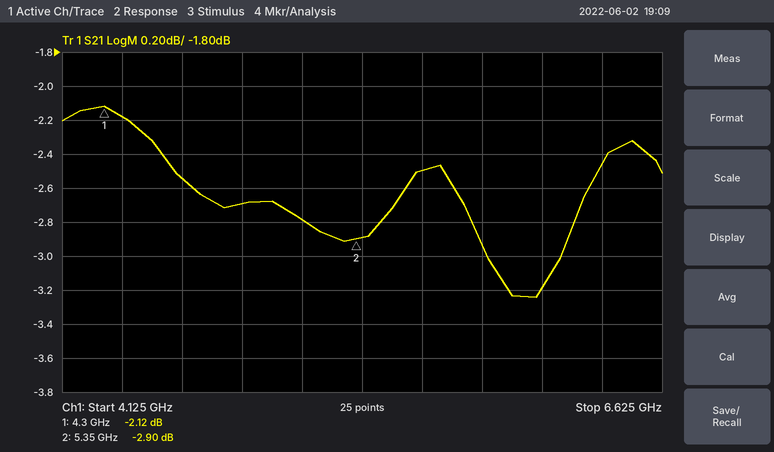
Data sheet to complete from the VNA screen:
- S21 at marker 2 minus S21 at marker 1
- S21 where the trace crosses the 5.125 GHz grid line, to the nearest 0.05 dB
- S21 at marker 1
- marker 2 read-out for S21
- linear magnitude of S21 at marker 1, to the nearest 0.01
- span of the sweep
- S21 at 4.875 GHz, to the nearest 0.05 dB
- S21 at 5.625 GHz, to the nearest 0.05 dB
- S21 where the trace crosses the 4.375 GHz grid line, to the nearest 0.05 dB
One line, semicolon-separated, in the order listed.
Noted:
-0.78 dB; -2.80 dB; -2.12 dB; -2.90 dB; 0.78; 2.5 GHz; -2.70 dB; -2.50 dB; -2.20 dB
